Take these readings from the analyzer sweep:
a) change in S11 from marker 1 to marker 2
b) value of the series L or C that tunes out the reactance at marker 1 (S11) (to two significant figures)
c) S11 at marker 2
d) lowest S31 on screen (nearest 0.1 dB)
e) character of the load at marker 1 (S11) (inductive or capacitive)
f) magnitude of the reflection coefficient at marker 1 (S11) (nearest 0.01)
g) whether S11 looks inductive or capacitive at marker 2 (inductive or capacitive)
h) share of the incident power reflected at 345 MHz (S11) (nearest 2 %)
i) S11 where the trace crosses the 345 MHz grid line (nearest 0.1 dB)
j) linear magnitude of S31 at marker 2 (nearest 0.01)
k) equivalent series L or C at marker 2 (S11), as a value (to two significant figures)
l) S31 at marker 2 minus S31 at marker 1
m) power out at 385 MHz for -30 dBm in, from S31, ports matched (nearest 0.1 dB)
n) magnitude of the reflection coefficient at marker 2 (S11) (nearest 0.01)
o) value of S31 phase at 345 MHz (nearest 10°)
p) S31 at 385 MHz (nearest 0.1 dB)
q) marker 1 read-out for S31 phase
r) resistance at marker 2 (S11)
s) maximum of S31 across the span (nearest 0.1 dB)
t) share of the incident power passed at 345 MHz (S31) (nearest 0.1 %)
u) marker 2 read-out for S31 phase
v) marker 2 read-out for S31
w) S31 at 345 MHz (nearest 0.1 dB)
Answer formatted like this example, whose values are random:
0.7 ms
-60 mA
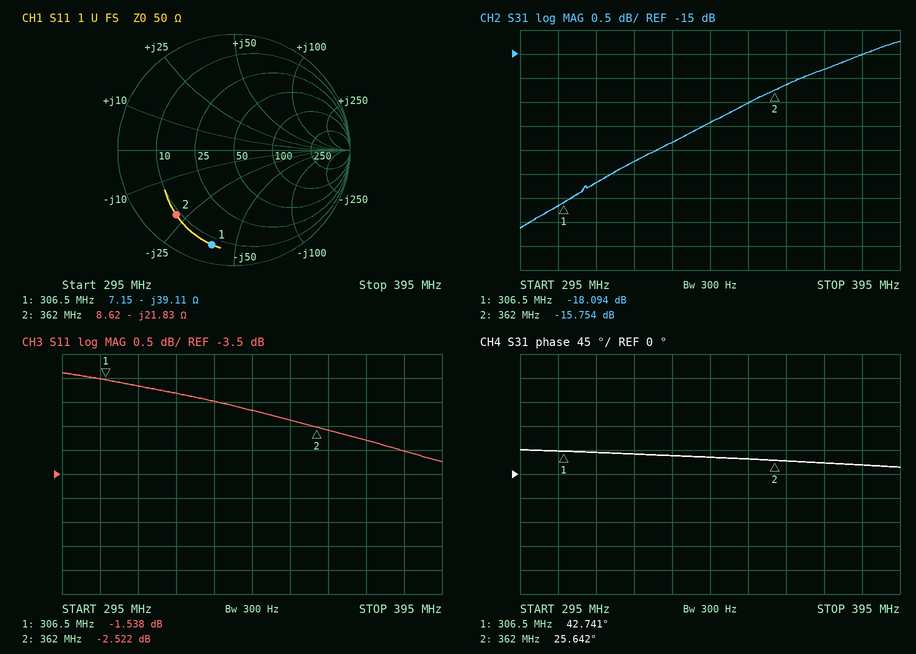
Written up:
-0.984 dB
20 nH
-2.522 dB
-18.6 dB
capacitive
0.84
capacitive
60 %
-2.2 dB
0.16
20 pF
2.340 dB
-45.0 dBm
0.75
30°
-15.0 dB
42.741°
8.62 Ω
-14.7 dB
2.3 %
25.642°
-15.754 dB
-16.4 dB
